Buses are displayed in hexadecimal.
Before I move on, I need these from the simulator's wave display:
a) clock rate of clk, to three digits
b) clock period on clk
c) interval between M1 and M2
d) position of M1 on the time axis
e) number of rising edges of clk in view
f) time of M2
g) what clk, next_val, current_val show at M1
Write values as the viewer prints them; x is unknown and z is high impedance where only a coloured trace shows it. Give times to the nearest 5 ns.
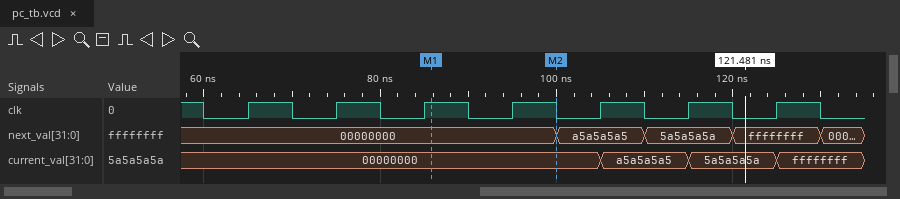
100 MHz
10 ns
15 ns
85 ns
7
100 ns
clk=1, next_val=00000000, current_val=00000000
